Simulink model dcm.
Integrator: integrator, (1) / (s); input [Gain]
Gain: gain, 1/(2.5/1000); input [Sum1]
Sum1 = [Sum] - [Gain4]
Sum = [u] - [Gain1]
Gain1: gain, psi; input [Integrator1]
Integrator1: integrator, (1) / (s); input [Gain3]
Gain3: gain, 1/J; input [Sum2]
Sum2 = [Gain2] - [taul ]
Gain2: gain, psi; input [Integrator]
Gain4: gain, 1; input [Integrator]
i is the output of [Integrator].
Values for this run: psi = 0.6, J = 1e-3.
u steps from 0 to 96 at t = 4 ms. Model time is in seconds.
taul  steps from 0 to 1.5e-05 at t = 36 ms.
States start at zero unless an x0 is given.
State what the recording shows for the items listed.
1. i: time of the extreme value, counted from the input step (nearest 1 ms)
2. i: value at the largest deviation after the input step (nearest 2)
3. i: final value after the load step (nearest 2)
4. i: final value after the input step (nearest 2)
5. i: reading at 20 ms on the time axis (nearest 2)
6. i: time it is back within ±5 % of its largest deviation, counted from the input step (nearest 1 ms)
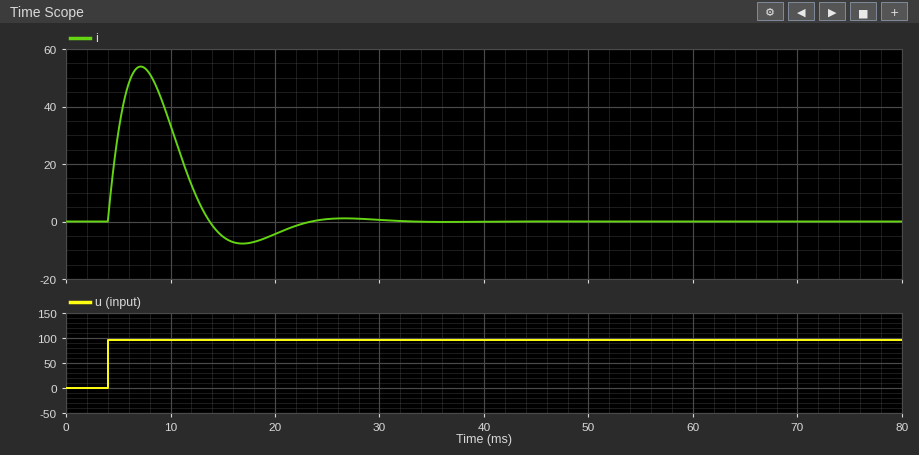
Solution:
3 ms
54
0
0
-4
17 ms
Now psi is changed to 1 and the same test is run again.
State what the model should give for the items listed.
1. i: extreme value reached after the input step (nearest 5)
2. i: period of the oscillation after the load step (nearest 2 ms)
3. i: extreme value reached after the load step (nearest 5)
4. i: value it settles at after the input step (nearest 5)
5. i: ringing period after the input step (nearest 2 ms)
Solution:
40
10 ms
0
0
10 ms
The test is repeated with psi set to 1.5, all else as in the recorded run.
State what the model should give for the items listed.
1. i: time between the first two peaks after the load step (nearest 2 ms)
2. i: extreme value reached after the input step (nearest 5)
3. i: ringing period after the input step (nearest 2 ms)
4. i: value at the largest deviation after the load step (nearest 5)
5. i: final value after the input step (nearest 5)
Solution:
6 ms
30
6 ms
0
0
